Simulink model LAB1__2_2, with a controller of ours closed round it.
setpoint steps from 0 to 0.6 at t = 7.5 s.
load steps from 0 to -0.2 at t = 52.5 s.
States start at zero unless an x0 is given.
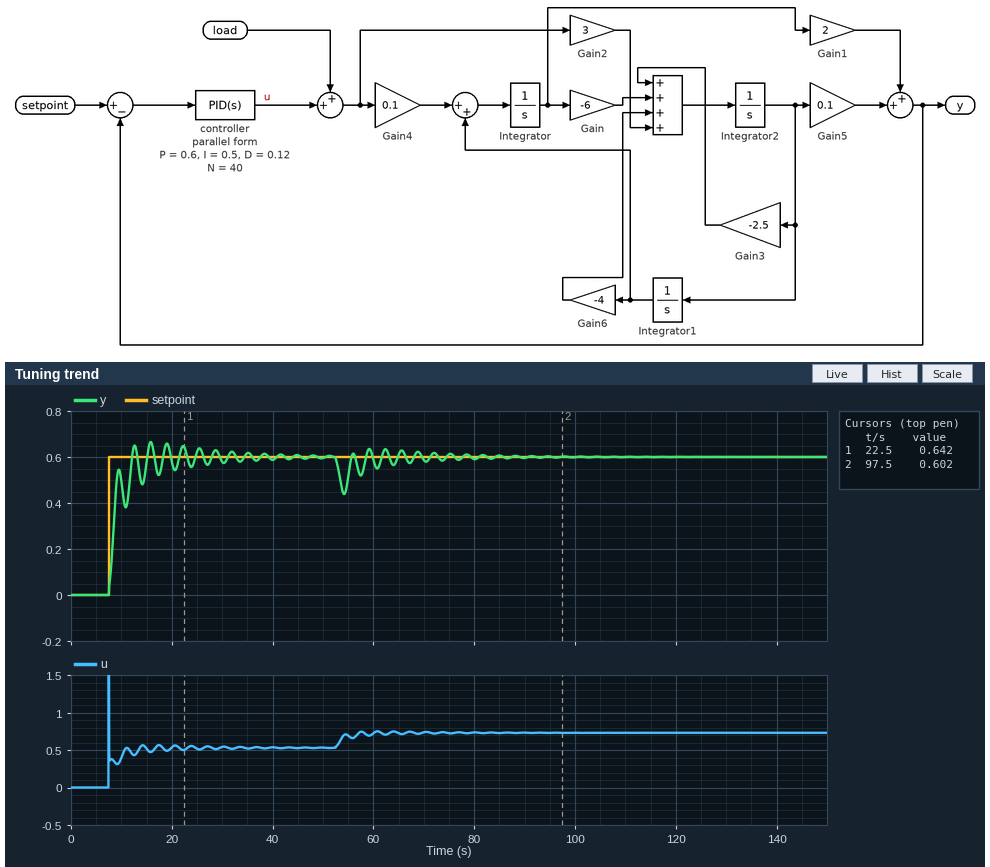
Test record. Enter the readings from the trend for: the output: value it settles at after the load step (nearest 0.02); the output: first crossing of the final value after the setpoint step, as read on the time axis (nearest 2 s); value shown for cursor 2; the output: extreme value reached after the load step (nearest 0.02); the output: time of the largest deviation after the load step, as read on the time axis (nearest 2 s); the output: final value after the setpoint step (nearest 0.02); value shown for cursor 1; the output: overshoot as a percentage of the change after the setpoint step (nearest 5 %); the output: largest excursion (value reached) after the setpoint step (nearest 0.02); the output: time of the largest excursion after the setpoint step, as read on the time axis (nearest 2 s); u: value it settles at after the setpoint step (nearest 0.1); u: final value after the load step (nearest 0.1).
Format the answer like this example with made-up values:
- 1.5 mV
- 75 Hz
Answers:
- 0.60
- 12 s
- 0.602
- 0.44
- 54 s
- 0.60
- 0.642
- 10 %
- 0.66
- 16 s
- 0.5
- 0.7
